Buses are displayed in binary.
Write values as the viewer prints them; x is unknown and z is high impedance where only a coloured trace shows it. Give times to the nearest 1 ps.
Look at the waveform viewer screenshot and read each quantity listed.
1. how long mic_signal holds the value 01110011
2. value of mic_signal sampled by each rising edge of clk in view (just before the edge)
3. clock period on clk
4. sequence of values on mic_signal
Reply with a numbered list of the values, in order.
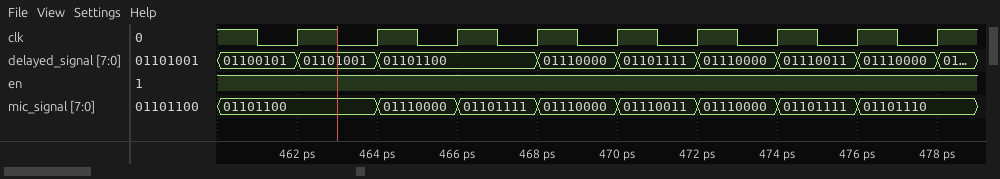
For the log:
1. 2 ps
2. 01101100, 01101100, 01110000, 01101111, 01110000, 01110011, 01110000, 01101111, 01101110
3. 2 ps
4. 01101100, 01110000, 01101111, 01110000, 01110011, 01110000, 01101111, 01101110
